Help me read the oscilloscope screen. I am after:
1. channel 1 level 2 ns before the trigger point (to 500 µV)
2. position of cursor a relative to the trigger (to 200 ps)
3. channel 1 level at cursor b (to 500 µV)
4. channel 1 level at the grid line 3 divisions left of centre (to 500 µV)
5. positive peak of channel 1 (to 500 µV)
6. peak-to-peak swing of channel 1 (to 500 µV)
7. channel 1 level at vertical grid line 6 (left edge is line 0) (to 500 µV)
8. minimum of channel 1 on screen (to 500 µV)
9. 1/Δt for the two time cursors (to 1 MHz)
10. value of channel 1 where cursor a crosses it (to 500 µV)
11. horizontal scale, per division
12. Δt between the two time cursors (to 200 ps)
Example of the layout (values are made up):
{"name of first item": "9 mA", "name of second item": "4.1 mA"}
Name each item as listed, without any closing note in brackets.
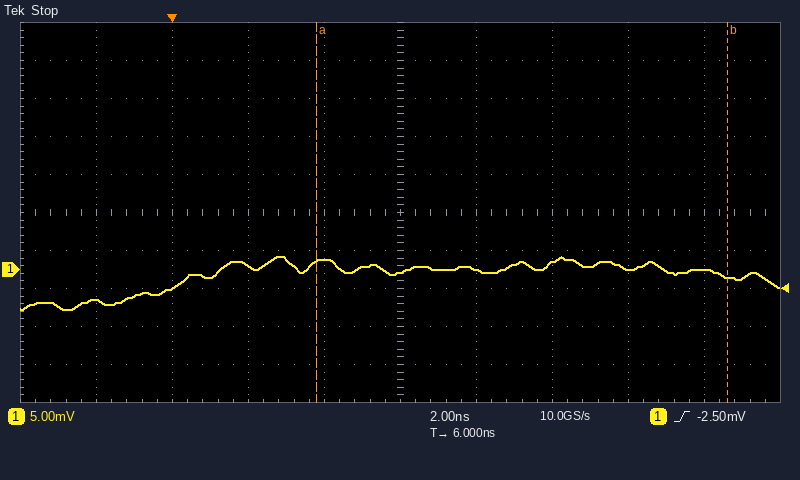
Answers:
{"channel 1 level 2 ns before the trigger point": "-4.0 mV", "position of cursor a relative to the trigger": "+3.8 ns", "channel 1 level at cursor b": "-1.0 mV", "channel 1 level at the grid line 3 divisions left of centre": "-2.5 mV", "positive peak of channel 1": "1.5 mV", "peak-to-peak swing of channel 1": "7.0 mV", "channel 1 level at vertical grid line 6 (left edge is line 0)": "0.0 mV", "minimum of channel 1 on screen": "-5.5 mV", "1/Δt for the two time cursors": "93 MHz", "value of channel 1 where cursor a crosses it": "1.0 mV", "horizontal scale, per division": "2 ns", "Δt between the two time cursors": "10.8 ns"}
